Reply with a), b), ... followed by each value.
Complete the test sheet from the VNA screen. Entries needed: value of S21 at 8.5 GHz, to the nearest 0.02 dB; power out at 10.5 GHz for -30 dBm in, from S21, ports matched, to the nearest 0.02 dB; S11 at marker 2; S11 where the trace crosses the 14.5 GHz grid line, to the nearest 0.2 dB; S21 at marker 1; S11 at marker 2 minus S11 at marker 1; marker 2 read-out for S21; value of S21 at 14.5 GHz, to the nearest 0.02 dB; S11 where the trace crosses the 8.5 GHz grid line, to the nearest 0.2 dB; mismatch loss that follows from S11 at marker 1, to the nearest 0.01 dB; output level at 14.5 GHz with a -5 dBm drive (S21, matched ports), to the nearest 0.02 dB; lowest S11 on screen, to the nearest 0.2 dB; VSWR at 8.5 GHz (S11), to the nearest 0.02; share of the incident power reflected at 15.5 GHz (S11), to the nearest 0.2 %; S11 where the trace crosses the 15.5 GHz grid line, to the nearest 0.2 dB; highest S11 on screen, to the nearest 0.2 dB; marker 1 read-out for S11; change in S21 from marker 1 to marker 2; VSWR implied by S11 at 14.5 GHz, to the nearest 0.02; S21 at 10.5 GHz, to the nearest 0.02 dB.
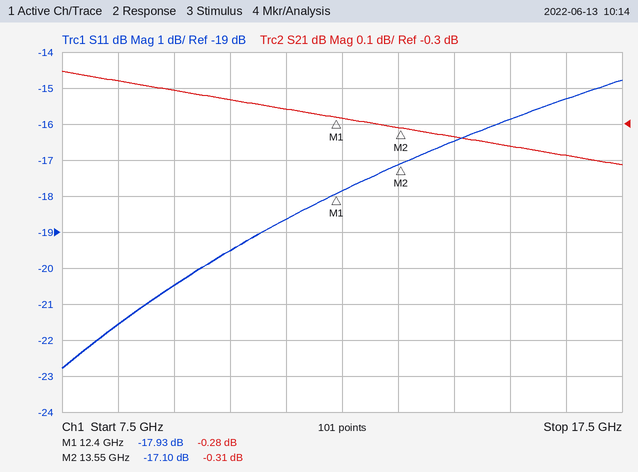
a) -0.18 dB
b) -30.24 dBm
c) -17.10 dB
d) -16.4 dB
e) -0.28 dB
f) 0.83 dB
g) -0.31 dB
h) -0.34 dB
i) -21.6 dB
j) 0.07 dB
k) -5.34 dBm
l) -22.8 dB
m) 1.18
n) 2.6 %
o) -15.8 dB
p) -14.8 dB
q) -17.93 dB
r) -0.03 dB
s) 1.36
t) -0.24 dB
